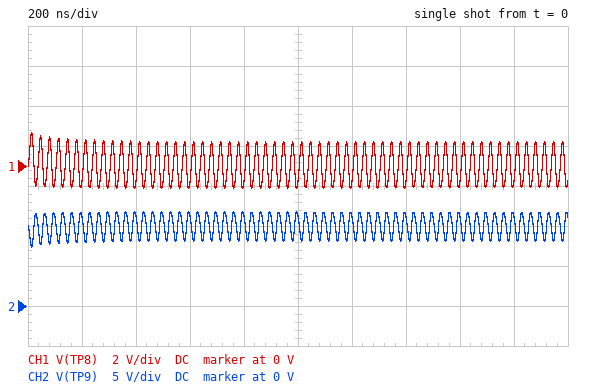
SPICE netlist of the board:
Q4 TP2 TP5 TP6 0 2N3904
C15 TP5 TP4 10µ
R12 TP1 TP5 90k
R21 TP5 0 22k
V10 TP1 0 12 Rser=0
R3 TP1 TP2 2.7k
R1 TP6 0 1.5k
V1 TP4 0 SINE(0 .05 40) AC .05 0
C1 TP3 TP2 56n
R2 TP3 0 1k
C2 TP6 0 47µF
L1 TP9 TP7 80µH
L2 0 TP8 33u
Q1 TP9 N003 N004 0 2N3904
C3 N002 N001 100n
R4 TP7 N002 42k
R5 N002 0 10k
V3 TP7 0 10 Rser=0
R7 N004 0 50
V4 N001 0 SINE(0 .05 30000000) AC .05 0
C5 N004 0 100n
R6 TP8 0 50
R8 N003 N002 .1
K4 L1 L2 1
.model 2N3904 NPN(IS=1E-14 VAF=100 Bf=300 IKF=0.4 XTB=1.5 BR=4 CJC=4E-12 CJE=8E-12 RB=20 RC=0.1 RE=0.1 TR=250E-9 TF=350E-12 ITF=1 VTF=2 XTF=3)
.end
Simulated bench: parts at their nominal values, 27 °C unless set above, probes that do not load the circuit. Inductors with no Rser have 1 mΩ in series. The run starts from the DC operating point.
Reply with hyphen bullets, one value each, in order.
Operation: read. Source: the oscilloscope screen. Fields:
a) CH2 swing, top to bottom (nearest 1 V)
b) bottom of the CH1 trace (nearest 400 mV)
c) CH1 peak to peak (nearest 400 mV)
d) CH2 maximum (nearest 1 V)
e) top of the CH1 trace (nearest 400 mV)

- 4 V
- -1.2 V
- 2.8 V
- 12 V
- 1.6 V
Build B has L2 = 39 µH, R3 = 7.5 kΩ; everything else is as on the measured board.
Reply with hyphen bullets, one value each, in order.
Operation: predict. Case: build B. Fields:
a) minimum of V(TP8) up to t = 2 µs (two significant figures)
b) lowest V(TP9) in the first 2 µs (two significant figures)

- -1.0 V
- 7.7 V
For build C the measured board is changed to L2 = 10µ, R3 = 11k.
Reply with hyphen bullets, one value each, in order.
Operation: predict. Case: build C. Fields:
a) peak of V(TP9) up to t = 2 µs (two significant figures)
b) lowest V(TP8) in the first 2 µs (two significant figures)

- 14 V
- -1.5 V
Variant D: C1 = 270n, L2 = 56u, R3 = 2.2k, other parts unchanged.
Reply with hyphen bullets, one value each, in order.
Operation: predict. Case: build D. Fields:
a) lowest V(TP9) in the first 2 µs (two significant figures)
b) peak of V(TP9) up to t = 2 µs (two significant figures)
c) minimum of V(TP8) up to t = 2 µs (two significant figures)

- 8.3 V
- 11 V
- -860 mV
